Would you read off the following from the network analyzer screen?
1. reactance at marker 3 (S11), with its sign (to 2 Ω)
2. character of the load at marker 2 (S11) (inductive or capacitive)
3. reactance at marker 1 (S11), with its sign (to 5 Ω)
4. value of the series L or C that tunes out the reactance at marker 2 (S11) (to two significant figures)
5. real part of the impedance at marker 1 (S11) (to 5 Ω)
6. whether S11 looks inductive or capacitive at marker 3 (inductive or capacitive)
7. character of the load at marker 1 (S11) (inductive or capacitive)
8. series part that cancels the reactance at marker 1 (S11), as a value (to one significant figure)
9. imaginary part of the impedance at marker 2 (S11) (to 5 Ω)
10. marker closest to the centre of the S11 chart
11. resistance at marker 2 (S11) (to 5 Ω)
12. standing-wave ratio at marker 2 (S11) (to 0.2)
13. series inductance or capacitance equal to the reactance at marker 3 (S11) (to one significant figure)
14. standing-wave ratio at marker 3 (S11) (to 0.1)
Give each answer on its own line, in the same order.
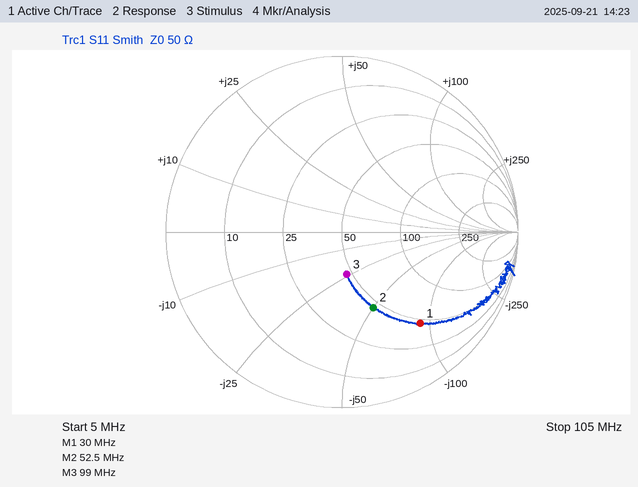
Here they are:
-24 Ω
capacitive
-90 Ω
150 nH
45 Ω
capacitive
capacitive
500 nH
-50 Ω
marker 3
45 Ω
2.8
70 pF
1.6
